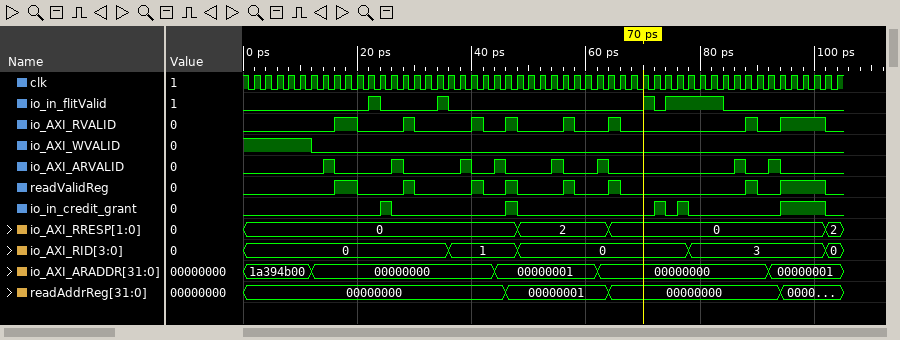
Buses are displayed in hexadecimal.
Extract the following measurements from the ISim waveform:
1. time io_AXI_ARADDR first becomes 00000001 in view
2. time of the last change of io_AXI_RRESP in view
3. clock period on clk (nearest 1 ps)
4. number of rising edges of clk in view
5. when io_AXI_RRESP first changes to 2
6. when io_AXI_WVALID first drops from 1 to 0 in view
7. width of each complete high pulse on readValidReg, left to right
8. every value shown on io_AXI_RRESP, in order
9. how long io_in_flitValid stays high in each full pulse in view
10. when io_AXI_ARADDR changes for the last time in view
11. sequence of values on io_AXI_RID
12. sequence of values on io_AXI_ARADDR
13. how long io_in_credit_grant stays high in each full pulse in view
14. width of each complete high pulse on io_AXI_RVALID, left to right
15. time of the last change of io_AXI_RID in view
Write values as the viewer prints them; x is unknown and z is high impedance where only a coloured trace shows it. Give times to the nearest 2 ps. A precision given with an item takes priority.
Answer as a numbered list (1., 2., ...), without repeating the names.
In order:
1. 44 ps
2. 102 ps
3. 2 ps
4. 52
5. 48 ps
6. 12 ps
7. 4 ps, 2 ps, 2 ps, 2 ps, 2 ps, 2 ps, 2 ps, 8 ps
8. 0, 2, 0, 2
9. 2 ps, 2 ps, 2 ps, 10 ps
10. 92 ps
11. 0, 1, 0, 3, 0
12. 1a394b00, 00000000, 00000001, 00000000, 00000001
13. 2 ps, 2 ps, 2 ps, 2 ps, 8 ps
14. 4 ps, 2 ps, 2 ps, 2 ps, 2 ps, 2 ps, 2 ps, 8 ps
15. 102 ps
